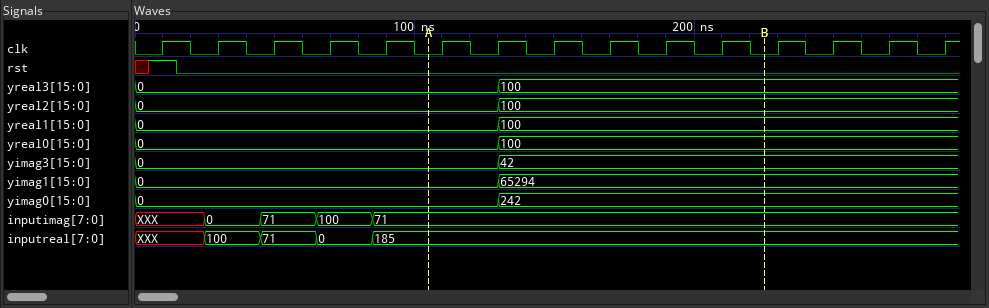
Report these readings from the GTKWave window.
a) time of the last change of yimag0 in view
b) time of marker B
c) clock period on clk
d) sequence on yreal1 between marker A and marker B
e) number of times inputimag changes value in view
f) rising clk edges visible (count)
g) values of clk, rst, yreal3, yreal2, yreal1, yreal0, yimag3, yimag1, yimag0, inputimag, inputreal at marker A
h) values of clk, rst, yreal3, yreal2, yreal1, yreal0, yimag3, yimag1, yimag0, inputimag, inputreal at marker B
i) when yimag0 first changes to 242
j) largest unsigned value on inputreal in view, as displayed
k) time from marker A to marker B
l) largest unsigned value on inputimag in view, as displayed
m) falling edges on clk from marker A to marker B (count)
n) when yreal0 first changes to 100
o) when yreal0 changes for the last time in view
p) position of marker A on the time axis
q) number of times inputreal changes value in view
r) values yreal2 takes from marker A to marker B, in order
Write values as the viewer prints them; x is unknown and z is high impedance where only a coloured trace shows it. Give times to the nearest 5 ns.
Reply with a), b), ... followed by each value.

a) 130 ns
b) 225 ns
c) 20 ns
d) 0, 100
e) 4
f) 15
g) clk=0, rst=0, yreal3=0, yreal2=0, yreal1=0, yreal0=0, yimag3=0, yimag1=0, yimag0=0, inputimag=71, inputreal=185
h) clk=0, rst=0, yreal3=100, yreal2=100, yreal1=100, yreal0=100, yimag3=42, yimag1=65294, yimag0=242, inputimag=71, inputreal=185
i) 130 ns
j) 185
k) 120 ns
l) 100
m) 6
n) 130 ns
o) 130 ns
p) 105 ns
q) 4
r) 0, 100
